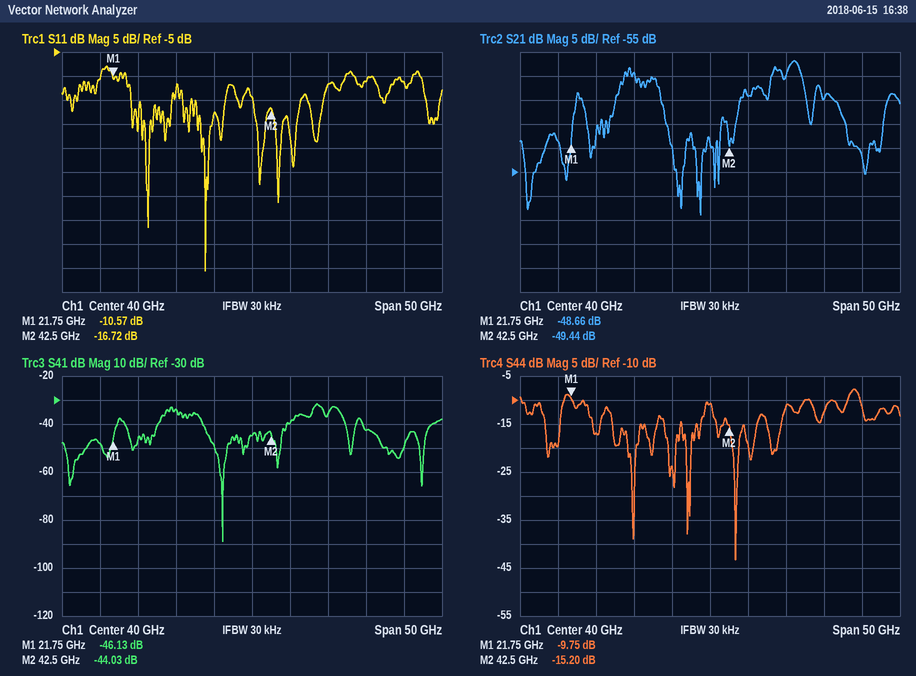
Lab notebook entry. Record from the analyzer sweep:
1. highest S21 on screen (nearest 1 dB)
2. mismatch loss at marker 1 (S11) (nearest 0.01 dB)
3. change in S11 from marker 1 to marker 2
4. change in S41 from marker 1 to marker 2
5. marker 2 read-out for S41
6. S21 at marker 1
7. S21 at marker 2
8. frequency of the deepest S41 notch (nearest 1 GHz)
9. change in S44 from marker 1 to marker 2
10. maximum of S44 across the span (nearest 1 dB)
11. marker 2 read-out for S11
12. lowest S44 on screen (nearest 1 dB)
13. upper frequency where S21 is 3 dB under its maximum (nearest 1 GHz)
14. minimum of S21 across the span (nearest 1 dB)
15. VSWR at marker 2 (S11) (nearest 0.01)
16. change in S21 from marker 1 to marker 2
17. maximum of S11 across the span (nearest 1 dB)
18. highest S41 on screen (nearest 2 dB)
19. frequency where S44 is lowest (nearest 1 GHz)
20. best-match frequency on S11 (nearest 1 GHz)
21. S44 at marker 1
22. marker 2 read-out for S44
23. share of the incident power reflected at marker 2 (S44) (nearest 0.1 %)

-32 dB
0.40 dB
-6.15 dB
2.10 dB
-44.03 dB
-48.66 dB
-49.44 dB
36 GHz
-5.45 dB
-8 dB
-16.72 dB
-43 dB
52 GHz
-64 dB
1.34
-0.78 dB
-8 dB
-32 dB
43 GHz
34 GHz
-9.75 dB
-15.20 dB
3.0 %
